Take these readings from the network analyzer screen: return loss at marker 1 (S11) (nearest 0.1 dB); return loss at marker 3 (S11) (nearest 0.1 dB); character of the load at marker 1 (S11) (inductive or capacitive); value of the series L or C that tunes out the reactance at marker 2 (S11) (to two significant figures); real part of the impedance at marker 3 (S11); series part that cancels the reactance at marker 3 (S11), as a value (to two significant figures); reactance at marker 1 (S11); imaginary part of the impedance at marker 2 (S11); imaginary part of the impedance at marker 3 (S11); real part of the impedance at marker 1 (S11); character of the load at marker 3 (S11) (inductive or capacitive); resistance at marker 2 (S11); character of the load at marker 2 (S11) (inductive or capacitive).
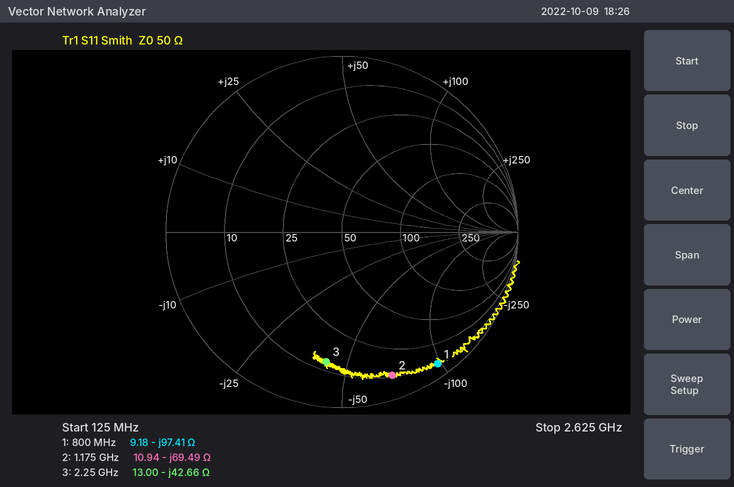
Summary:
0.7 dB
2.6 dB
capacitive
9.4 nH
13.00 Ω
3.0 nH
-97.41 Ω
-69.49 Ω
-42.66 Ω
9.18 Ω
capacitive
10.94 Ω
capacitive
